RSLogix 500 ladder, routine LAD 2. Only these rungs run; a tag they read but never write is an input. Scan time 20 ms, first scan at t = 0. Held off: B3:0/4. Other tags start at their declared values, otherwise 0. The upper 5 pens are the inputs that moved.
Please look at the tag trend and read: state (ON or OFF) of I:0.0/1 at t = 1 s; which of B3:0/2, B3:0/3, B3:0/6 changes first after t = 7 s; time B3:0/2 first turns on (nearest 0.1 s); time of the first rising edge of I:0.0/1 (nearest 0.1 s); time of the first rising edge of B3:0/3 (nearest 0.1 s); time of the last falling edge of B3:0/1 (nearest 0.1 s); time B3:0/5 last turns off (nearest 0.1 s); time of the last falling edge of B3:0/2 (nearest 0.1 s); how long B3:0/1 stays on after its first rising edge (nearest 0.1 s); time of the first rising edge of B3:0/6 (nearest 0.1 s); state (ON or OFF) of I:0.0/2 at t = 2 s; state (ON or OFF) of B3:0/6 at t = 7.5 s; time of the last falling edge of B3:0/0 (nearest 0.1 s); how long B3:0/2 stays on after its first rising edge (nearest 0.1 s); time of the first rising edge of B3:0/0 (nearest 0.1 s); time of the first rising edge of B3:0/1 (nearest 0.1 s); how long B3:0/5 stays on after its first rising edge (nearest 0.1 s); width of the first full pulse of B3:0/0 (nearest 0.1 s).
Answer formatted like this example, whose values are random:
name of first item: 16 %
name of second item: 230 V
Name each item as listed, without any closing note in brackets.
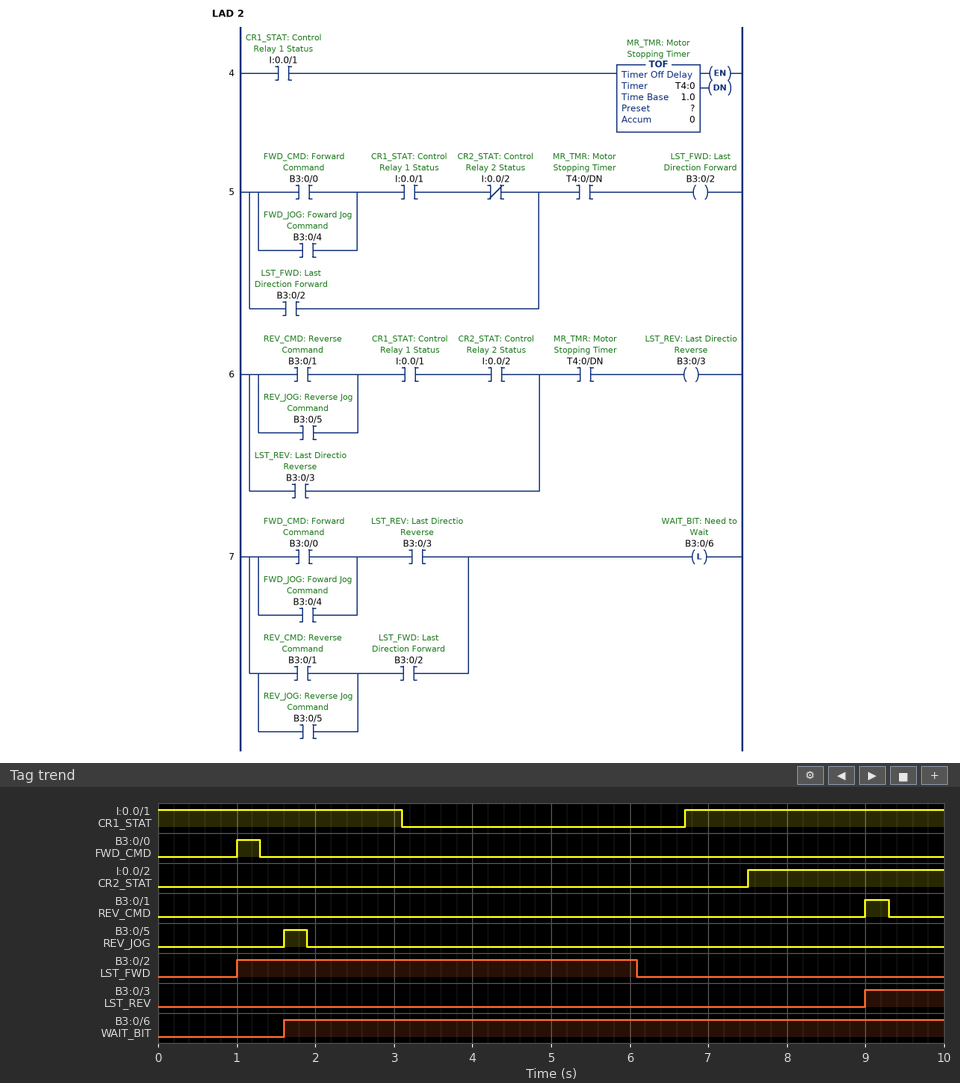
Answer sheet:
state (ON or OFF) of I:0.0/1 at t = 1 s: ON
which of B3:0/2, B3:0/3, B3:0/6 changes first after t = 7 s: B3:0/3
time B3:0/2 first turns on: 1.0 s
time of the first rising edge of I:0.0/1: 6.7 s
time of the first rising edge of B3:0/3: 9.0 s
time of the last falling edge of B3:0/1: 9.3 s
time B3:0/5 last turns off: 1.9 s
time of the last falling edge of B3:0/2: 6.1 s
how long B3:0/1 stays on after its first rising edge: 0.3 s
time of the first rising edge of B3:0/6: 1.6 s
state (ON or OFF) of I:0.0/2 at t = 2 s: OFF
state (ON or OFF) of B3:0/6 at t = 7.5 s: ON
time of the last falling edge of B3:0/0: 1.3 s
how long B3:0/2 stays on after its first rising edge: 5.1 s
time of the first rising edge of B3:0/0: 1.0 s
time of the first rising edge of B3:0/1: 9.0 s
how long B3:0/5 stays on after its first rising edge: 0.3 s
width of the first full pulse of B3:0/0: 0.3 s
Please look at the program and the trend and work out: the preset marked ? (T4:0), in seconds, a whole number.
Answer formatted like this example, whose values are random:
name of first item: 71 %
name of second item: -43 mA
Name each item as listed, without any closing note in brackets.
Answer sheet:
the preset marked ? (T4:0), in seconds, a whole number: 3 s
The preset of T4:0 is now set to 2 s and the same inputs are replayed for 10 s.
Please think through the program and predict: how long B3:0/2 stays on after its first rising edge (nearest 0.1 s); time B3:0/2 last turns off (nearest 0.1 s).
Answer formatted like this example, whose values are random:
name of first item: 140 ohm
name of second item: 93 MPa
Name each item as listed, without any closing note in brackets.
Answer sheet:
how long B3:0/2 stays on after its first rising edge: 4.1 s
time B3:0/2 last turns off: 5.1 s
